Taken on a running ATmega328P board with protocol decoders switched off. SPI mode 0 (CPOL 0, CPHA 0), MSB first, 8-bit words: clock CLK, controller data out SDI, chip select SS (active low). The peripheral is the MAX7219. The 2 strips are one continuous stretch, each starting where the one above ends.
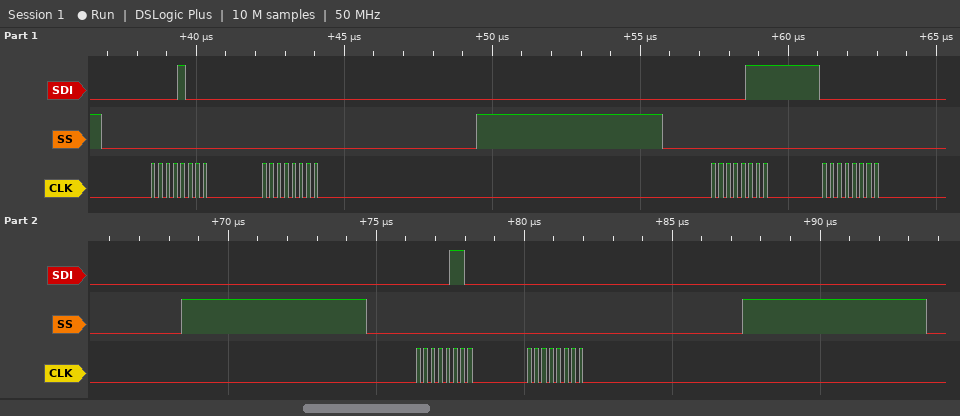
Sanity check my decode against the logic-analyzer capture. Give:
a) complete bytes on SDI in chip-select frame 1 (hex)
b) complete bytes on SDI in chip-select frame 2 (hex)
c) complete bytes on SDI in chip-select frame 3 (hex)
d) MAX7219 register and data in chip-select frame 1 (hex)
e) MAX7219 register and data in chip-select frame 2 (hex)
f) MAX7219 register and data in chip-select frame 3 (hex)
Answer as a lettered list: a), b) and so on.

a) 0x08 0x00
b) 0x07 0x00
c) 0x06 0x00
d) register 0x8, data 0x00
e) register 0x7, data 0x00
f) register 0x6, data 0x00
